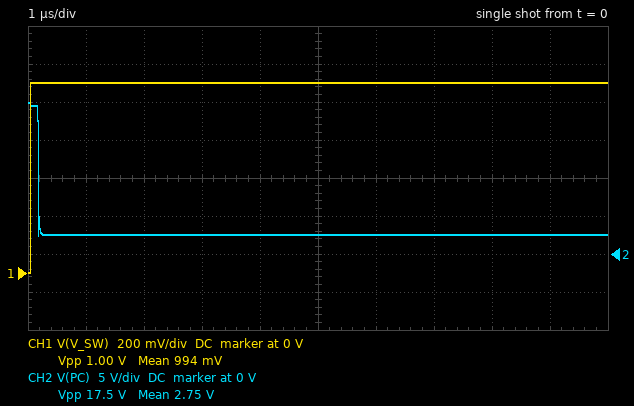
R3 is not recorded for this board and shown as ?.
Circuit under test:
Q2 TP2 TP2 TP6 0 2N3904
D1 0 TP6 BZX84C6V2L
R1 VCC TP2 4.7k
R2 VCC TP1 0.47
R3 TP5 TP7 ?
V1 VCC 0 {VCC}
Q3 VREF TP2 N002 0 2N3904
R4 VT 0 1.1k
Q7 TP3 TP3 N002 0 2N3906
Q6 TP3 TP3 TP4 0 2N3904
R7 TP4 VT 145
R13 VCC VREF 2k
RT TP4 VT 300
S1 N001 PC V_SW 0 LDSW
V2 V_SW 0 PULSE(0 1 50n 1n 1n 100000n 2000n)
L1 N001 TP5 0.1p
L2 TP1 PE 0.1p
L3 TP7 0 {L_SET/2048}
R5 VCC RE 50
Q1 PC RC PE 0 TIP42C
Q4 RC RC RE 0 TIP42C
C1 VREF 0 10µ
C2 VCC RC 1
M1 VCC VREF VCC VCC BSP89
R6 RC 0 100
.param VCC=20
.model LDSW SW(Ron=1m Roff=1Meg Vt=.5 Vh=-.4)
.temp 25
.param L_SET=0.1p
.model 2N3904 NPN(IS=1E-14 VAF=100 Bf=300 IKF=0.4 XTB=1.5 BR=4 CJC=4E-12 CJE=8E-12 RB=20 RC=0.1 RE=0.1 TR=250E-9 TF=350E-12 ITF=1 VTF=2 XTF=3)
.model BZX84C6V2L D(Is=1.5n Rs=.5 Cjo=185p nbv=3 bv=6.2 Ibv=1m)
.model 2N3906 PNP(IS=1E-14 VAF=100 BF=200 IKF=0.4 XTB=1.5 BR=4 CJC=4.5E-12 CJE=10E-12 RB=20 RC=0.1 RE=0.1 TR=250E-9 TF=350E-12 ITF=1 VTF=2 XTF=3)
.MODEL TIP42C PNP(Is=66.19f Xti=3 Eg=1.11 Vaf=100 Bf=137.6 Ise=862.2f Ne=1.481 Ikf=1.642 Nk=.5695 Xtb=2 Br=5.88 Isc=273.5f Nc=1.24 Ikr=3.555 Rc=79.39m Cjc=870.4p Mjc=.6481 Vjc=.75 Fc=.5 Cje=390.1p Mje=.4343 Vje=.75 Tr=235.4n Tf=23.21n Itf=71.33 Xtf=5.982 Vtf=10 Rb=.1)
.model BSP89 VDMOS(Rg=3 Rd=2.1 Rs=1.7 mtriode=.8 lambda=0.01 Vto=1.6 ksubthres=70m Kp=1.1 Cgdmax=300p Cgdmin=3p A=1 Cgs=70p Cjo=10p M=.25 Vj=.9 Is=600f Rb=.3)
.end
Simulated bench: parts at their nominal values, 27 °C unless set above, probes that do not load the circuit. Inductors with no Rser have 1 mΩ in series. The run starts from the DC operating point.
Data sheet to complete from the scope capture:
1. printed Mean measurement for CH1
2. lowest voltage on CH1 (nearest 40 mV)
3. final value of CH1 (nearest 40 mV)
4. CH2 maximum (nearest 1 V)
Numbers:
994 mV
0 V
1.00 V
20 V
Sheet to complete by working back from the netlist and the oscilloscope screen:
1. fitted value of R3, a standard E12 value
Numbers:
8.2 Ω
